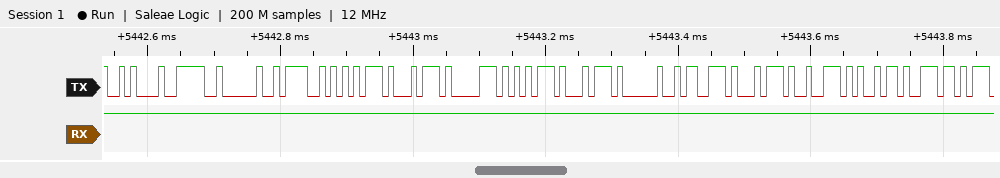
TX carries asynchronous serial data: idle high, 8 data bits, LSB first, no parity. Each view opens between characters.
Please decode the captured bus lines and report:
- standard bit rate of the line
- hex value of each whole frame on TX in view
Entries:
115200 baud
0A, 3E, 20, 4F, 75, 74, 70, 75, 74, 20, 73, 74, 72, 69, 6E
